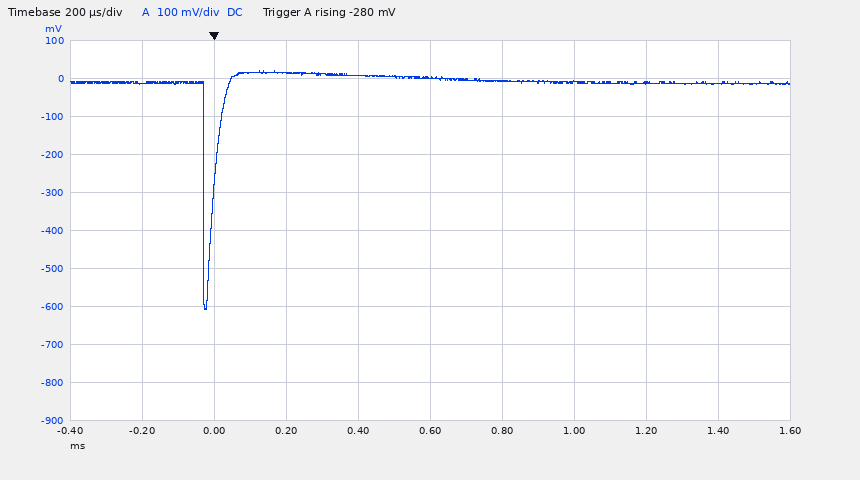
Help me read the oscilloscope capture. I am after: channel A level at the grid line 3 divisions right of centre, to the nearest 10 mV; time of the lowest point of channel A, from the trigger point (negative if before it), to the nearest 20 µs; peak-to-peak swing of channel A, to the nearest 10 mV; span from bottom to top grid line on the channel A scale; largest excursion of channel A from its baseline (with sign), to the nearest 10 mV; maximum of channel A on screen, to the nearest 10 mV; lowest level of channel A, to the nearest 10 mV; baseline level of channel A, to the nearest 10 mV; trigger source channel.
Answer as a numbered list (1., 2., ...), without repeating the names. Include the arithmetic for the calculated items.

1. -10 mV
2. -20 µs
3. 20 mV − (-610 mV) = 630 mV
4. 1 V
5. -610 mV − (-10 mV) = -600 mV
6. 20 mV
7. -610 mV
8. -10 mV
9. channel A
